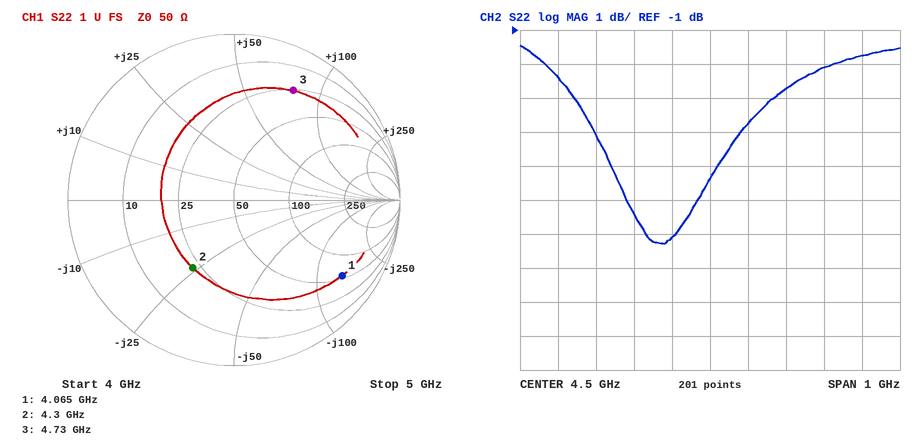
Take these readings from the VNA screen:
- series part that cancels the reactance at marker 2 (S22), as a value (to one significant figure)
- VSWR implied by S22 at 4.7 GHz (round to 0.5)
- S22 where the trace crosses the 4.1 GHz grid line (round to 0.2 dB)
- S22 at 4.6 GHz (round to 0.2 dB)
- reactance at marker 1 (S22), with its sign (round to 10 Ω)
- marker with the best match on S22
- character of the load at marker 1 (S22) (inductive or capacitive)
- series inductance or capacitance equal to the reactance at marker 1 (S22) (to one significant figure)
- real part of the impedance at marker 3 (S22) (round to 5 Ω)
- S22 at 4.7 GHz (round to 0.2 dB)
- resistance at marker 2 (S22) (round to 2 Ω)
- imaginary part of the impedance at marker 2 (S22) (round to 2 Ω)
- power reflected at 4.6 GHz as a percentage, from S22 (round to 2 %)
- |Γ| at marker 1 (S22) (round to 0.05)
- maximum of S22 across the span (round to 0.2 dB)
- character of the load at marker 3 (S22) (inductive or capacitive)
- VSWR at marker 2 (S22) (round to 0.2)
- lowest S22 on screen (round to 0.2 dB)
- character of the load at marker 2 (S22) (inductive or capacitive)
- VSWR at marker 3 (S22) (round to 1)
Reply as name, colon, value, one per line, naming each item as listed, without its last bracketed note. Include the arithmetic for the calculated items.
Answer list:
series part that cancels the reactance at marker 2 (S22), as a value: L = 24 Ω/(2π × 4.3 GHz) ≈ 888 pH, so 900 pH to one significant figure
VSWR implied by S22 at 4.7 GHz: |Γ| = 10^(-2.8/20) = 0.7244; VSWR = (1 + 0.7244)/(1 − 0.7244) ≈ 6.26, so 6.5 to the nearest 0.5
S22 where the trace crosses the 4.1 GHz grid line: -2.4 dB
S22 at 4.6 GHz: -3.8 dB
reactance at marker 1 (S22), with its sign: -140 Ω
marker with the best match on S22: marker 2
character of the load at marker 1 (S22): capacitive
series inductance or capacitance equal to the reactance at marker 1 (S22): C = 1/(2π × 4.065 GHz × 140 Ω) ≈ 280 fF, so 300 fF to one significant figure
real part of the impedance at marker 3 (S22): 25 Ω
S22 at 4.7 GHz: -2.8 dB
resistance at marker 2 (S22): 22 Ω
imaginary part of the impedance at marker 2 (S22): -24 Ω
power reflected at 4.6 GHz as a percentage, from S22: 10^(-3.8/10) ≈ 42 %
|Γ| at marker 1 (S22): 0.80
maximum of S22 across the span: -1.4 dB
character of the load at marker 3 (S22): inductive
VSWR at marker 2 (S22): 2.8
lowest S22 on screen: -7.2 dB
character of the load at marker 2 (S22): capacitive
VSWR at marker 3 (S22): 7
